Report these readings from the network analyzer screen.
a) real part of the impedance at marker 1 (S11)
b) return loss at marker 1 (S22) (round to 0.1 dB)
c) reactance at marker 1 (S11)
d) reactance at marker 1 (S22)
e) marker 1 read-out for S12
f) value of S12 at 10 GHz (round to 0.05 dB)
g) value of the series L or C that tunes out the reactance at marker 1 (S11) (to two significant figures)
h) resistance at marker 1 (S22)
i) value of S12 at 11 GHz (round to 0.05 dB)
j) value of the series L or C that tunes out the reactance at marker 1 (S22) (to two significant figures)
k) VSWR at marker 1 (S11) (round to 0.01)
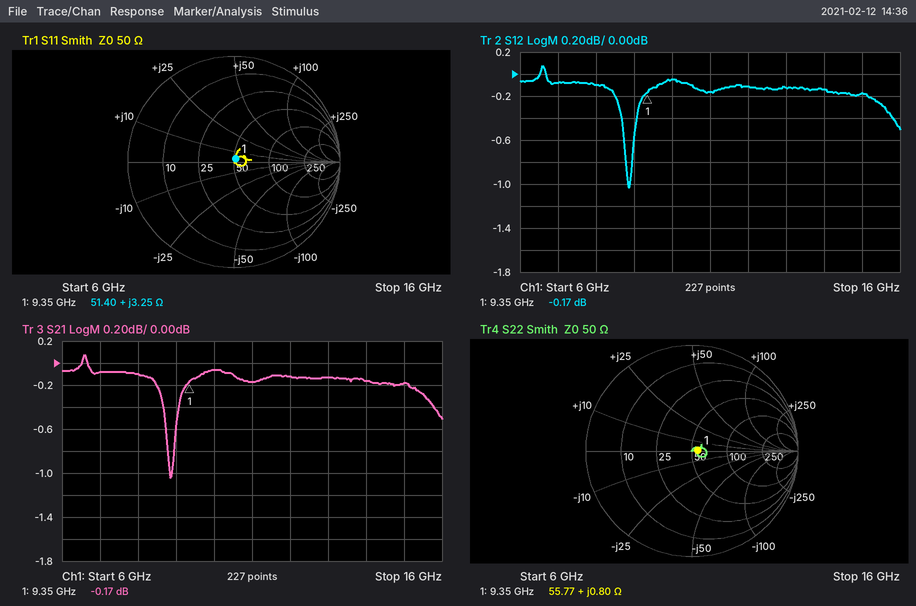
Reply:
51.40 Ω
25.2 dB
+3.25 Ω
+0.80 Ω
-0.17 dB
-0.05 dB
5.2 pF
55.77 Ω
-0.15 dB
21 pF
1.07
